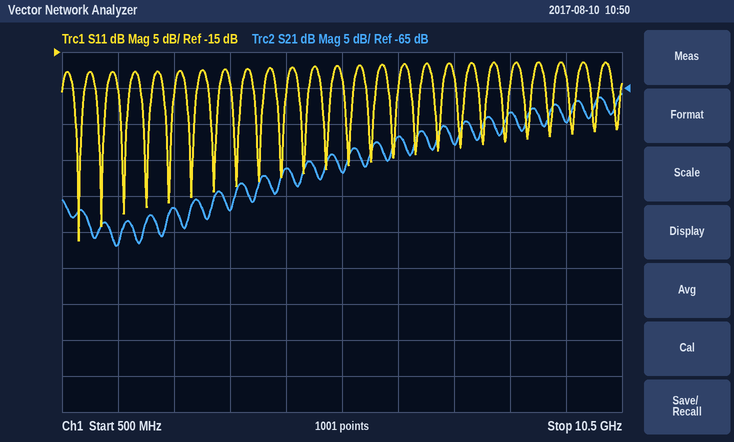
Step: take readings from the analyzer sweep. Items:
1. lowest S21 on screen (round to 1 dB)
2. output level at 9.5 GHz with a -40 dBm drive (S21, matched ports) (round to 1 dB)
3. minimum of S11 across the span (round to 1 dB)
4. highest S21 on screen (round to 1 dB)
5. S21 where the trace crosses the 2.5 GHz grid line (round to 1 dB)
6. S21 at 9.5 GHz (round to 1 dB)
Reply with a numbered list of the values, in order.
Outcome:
1. -87 dB
2. -110 dBm
3. -41 dB
4. -66 dB
5. -82 dB
6. -70 dB
